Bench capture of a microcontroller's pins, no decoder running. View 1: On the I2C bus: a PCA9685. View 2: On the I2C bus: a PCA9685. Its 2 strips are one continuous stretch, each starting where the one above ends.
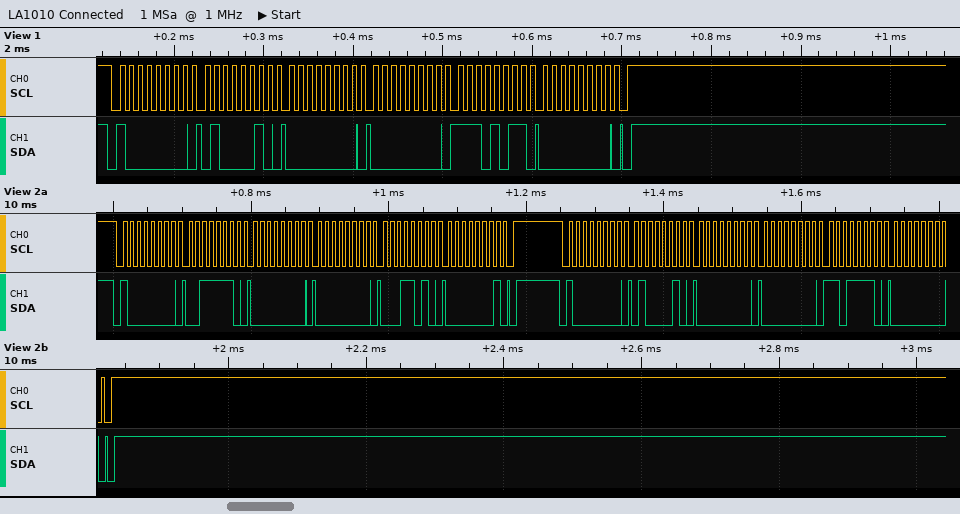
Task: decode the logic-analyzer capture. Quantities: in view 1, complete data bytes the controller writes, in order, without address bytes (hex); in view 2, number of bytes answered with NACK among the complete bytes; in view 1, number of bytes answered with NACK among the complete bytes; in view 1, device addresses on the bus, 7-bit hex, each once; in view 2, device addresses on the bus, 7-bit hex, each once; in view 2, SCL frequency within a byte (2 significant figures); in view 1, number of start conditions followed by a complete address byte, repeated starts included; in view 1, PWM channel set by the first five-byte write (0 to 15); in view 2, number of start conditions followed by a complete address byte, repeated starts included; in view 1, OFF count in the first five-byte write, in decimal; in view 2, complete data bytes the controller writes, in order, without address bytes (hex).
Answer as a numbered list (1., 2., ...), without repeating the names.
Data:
1. 42 00 00 EB 00
2. 0
3. 0
4. 0x40
5. 0x40
6. 100 kHz
7. 1
8. 15
9. 2
10. 235
11. 3E 00 00 1A 01 42 00 00 DE 00
